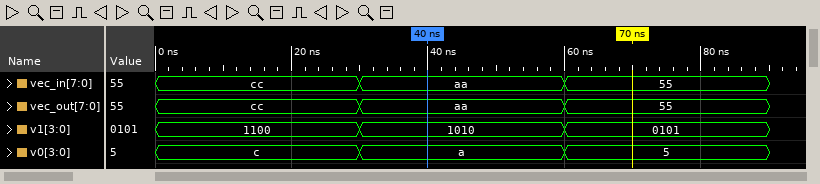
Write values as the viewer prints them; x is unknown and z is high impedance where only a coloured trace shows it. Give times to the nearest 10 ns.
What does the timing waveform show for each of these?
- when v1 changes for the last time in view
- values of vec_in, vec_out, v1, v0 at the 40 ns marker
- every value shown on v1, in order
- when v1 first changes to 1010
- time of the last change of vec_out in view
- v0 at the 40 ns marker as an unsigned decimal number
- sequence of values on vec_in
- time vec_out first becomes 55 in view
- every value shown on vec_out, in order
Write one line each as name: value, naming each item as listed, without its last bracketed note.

when v1 changes for the last time in view: 60 ns
values of vec_in, vec_out, v1, v0 at the 40 ns marker: vec_in=aa, vec_out=aa, v1=1010, v0=a
every value shown on v1, in order: 1100, 1010, 0101
when v1 first changes to 1010: 30 ns
time of the last change of vec_out in view: 60 ns
v0 at the 40 ns marker as an unsigned decimal number: 10
sequence of values on vec_in: cc, aa, 55
time vec_out first becomes 55 in view: 60 ns
every value shown on vec_out, in order: cc, aa, 55
